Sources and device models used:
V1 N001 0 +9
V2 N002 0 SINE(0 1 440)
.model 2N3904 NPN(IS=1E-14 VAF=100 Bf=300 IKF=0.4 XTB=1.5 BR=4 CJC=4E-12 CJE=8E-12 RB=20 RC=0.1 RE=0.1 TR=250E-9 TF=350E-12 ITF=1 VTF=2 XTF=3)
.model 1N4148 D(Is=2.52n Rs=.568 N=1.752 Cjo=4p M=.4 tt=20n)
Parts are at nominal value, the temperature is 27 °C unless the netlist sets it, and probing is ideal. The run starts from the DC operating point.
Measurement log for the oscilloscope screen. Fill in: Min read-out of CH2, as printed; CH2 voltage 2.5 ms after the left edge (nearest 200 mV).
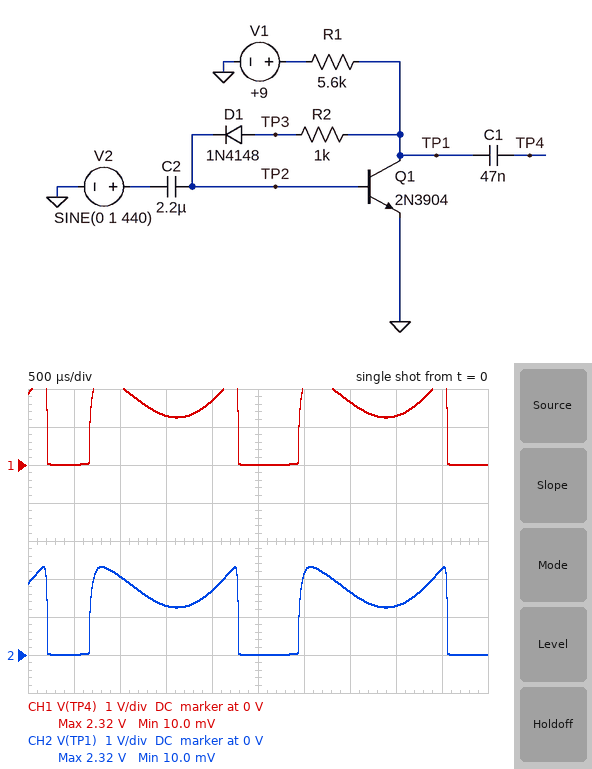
10.0 mV
0 V
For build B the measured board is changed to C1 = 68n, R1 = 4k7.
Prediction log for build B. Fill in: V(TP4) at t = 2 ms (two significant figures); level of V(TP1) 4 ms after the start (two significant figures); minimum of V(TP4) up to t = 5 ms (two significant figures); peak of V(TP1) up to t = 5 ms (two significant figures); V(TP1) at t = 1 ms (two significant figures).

2.0 V
1.6 V
9.0 mV
2.5 V
2.3 V
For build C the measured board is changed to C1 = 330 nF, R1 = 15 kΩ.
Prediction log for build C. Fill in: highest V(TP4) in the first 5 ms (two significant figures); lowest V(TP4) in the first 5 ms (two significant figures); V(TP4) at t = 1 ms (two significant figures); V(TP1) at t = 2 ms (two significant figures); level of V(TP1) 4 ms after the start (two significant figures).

1.6 V
7.4 mV
1.2 V
470 mV
110 mV
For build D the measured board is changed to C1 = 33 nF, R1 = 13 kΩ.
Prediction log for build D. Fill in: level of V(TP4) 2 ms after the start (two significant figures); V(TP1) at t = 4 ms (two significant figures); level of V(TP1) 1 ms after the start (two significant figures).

600 mV
230 mV
1.3 V
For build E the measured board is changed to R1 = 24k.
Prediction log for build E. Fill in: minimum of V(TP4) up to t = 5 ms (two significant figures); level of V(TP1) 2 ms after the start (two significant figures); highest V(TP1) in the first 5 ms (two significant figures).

-220 mV
130 mV
1.4 V
